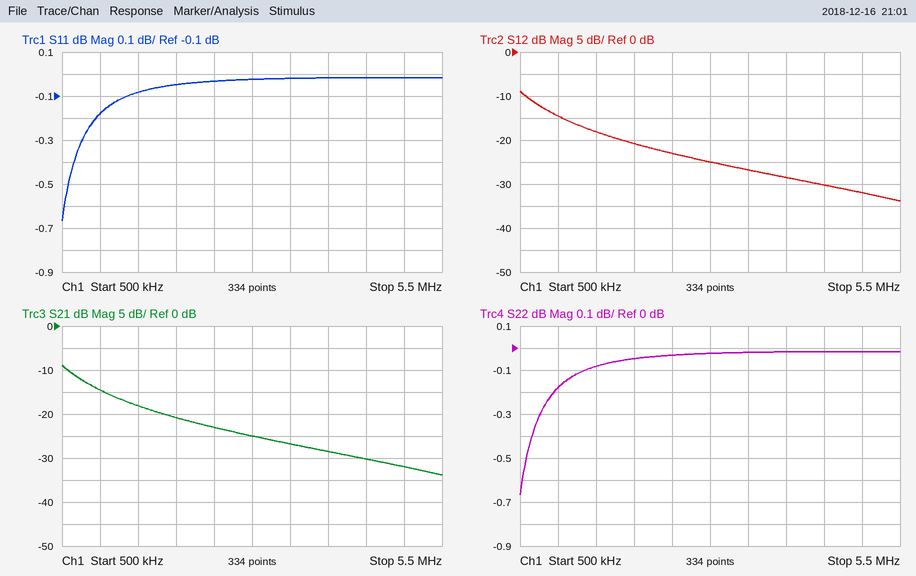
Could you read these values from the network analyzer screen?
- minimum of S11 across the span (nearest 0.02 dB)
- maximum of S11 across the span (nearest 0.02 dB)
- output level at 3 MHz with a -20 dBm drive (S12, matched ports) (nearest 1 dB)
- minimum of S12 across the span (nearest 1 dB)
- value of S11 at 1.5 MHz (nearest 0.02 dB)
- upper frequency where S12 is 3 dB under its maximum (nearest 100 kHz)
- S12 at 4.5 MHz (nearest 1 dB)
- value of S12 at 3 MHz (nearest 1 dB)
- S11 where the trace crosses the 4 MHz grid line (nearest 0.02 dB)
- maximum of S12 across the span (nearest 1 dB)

-0.66 dB
-0.02 dB
-45 dBm
-34 dB
-0.08 dB
700 kHz
-30 dB
-25 dB
-0.02 dB
-9 dB
